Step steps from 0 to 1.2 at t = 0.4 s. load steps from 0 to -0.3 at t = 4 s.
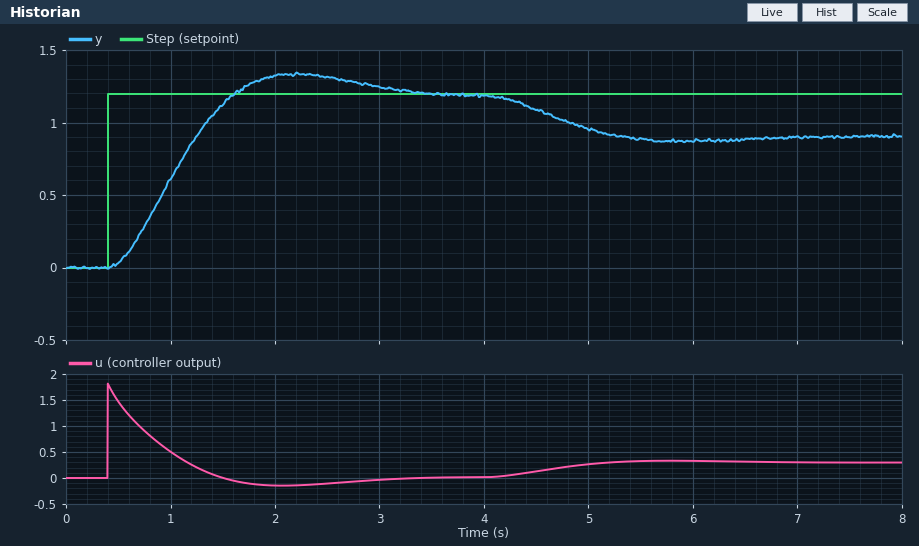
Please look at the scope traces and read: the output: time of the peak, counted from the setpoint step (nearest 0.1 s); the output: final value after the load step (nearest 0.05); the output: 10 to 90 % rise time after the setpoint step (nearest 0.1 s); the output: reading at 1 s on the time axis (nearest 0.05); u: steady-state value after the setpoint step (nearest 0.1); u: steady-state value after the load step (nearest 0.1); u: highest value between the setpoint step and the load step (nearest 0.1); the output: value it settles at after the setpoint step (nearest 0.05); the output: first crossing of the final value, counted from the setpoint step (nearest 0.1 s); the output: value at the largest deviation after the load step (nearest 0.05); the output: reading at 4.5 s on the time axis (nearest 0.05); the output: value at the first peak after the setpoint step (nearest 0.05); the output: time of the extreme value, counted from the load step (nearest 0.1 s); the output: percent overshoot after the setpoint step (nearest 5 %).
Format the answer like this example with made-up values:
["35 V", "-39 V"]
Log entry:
["1.8 s", "0.90", "0.8 s", "0.60", "0.0", "0.3", "1.8", "1.20", "1.2 s", "0.85", "1.10", "1.35", "1.9 s", "10 %"]
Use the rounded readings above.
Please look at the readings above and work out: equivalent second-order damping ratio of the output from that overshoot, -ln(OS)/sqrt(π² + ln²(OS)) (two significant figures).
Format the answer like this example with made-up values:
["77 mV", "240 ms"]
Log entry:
["0.59"]
